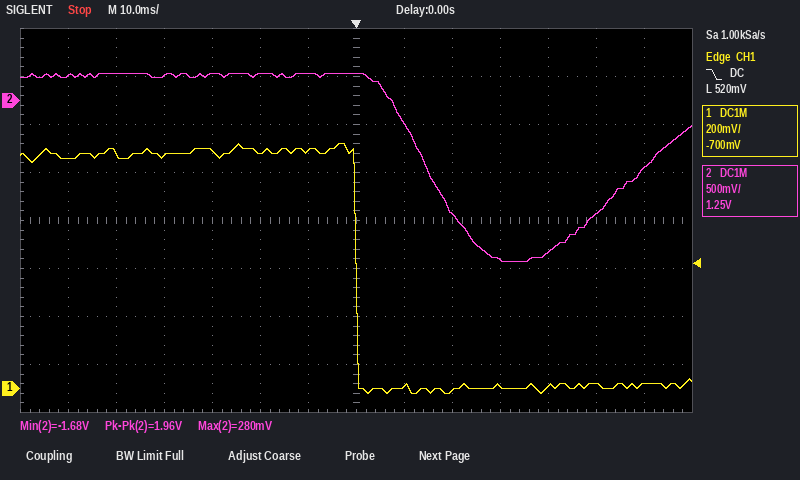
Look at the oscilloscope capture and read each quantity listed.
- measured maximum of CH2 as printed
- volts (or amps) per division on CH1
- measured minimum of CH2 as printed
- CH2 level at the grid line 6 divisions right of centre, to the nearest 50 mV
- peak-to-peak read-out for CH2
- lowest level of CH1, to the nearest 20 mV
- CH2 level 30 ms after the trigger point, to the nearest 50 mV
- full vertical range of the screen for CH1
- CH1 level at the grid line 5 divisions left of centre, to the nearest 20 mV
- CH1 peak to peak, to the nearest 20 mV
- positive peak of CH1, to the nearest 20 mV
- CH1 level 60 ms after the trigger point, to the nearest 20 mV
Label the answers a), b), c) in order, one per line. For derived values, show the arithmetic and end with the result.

a) 280 mV
b) 200 mV
c) -1.68 V
d) -700 mV
e) 1.96 V
f) -20 mV
g) -1.65 V
h) 1.6 V
i) 980 mV
j) 1.02 V − (-20 mV) = 1.04 V
k) 1.02 V
l) 20 mV
